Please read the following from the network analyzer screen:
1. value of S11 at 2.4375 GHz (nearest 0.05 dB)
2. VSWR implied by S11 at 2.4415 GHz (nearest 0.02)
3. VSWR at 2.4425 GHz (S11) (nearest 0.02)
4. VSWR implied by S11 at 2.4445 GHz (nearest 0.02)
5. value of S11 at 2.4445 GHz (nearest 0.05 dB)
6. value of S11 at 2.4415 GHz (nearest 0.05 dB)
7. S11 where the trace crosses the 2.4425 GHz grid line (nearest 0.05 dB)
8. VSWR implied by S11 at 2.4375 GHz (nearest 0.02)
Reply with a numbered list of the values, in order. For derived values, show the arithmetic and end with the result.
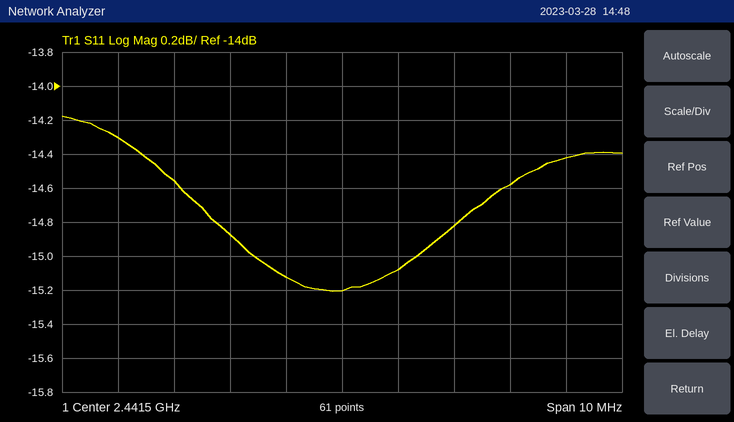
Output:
1. -14.30 dB
2. |Γ| = 10^(-15.2/20) = 0.1738; VSWR = (1 + 0.1738)/(1 − 0.1738) ≈ 1.42
3. |Γ| = 10^(-15.1/20) = 0.1758; VSWR = (1 + 0.1758)/(1 − 0.1758) ≈ 1.43, so 1.42 to the nearest 0.02
4. |Γ| = 10^(-14.6/20) = 0.1862; VSWR = (1 + 0.1862)/(1 − 0.1862) ≈ 1.46
5. -14.60 dB
6. -15.20 dB
7. -15.10 dB
8. |Γ| = 10^(-14.3/20) = 0.1928; VSWR = (1 + 0.1928)/(1 − 0.1928) ≈ 1.48
